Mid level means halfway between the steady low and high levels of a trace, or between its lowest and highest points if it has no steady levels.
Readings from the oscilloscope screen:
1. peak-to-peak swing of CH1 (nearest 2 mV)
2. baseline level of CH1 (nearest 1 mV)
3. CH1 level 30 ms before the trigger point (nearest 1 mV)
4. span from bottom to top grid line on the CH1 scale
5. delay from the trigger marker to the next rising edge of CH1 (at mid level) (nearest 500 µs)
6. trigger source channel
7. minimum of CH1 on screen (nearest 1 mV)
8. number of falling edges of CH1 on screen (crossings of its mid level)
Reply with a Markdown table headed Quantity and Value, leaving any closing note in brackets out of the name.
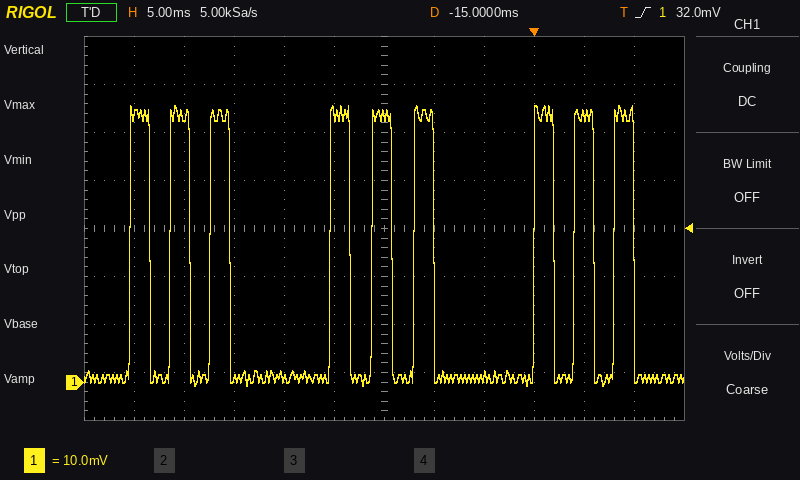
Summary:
| Quantity | Value |
|---|---|
| peak-to-peak swing of CH1 | 58 mV |
| baseline level of CH1 | 1 mV |
| CH1 level 30 ms before the trigger point | 1 mV |
| span from bottom to top grid line on the CH1 scale | 80 mV |
| delay from the trigger marker to the next rising edge of CH1 (at mid level) | 4.0 ms |
| trigger source channel | CH1 |
| minimum of CH1 on screen | -1 mV |
| number of falling edges of CH1 on screen | 9 |
